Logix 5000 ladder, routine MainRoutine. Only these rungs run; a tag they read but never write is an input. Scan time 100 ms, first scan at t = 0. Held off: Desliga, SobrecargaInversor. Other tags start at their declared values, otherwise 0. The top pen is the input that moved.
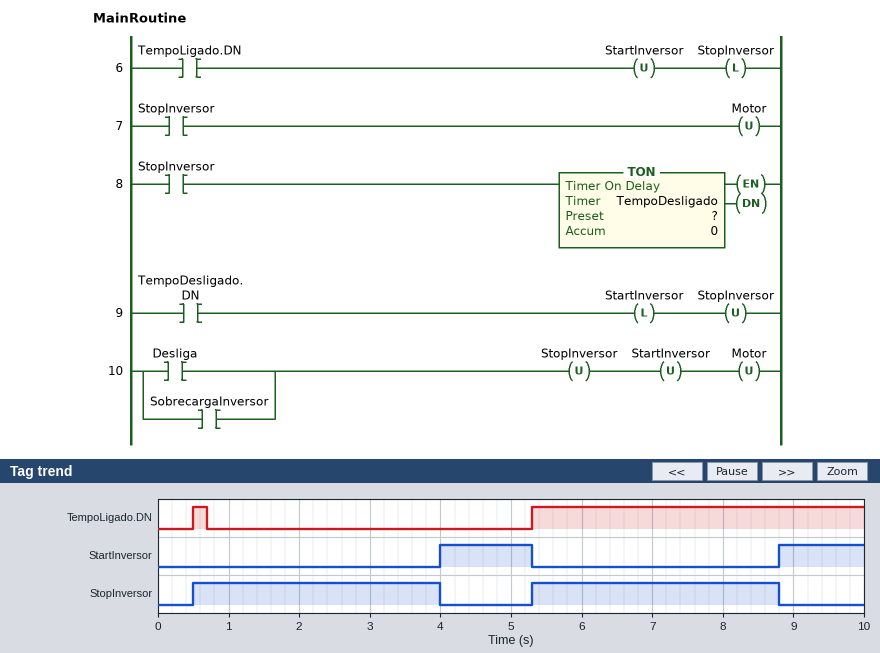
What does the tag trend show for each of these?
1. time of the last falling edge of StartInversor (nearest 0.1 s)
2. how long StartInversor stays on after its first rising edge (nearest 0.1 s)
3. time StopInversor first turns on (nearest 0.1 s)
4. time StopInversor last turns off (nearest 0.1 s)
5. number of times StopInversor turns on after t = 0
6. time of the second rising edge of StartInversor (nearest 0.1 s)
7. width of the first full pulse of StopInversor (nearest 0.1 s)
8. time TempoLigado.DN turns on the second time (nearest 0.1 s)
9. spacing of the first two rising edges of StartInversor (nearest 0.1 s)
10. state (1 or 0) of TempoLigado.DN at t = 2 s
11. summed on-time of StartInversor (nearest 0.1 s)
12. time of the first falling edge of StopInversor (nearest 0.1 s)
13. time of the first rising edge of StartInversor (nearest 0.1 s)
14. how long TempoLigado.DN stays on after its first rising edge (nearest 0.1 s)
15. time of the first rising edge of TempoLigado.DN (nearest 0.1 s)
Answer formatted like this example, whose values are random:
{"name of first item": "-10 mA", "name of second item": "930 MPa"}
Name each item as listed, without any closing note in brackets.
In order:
{"time of the last falling edge of StartInversor": "5.3 s", "how long StartInversor stays on after its first rising edge": "1.3 s", "time StopInversor first turns on": "0.5 s", "time StopInversor last turns off": "8.8 s", "number of times StopInversor turns on after t = 0": "2", "time of the second rising edge of StartInversor": "8.8 s", "width of the first full pulse of StopInversor": "3.5 s", "time TempoLigado.DN turns on the second time": "5.3 s", "spacing of the first two rising edges of StartInversor": "4.8 s", "state (1 or 0) of TempoLigado.DN at t = 2 s": "0", "summed on-time of StartInversor": "2.5 s", "time of the first falling edge of StopInversor": "4.0 s", "time of the first rising edge of StartInversor": "4.0 s", "how long TempoLigado.DN stays on after its first rising edge": "0.2 s", "time of the first rising edge of TempoLigado.DN": "0.5 s"}
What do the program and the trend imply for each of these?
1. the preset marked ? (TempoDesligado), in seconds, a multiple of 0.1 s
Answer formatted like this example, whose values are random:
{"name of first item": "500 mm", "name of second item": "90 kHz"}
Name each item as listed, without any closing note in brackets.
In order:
{"the preset marked ? (TempoDesligado), in seconds, a multiple of 0.1 s": "3.5 s"}
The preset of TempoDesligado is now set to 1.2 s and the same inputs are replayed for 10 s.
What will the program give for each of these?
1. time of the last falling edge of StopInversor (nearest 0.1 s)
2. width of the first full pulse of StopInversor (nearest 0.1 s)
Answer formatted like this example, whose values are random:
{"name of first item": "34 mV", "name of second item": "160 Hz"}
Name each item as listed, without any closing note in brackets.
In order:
{"time of the last falling edge of StopInversor": "6.5 s", "width of the first full pulse of StopInversor": "1.2 s"}
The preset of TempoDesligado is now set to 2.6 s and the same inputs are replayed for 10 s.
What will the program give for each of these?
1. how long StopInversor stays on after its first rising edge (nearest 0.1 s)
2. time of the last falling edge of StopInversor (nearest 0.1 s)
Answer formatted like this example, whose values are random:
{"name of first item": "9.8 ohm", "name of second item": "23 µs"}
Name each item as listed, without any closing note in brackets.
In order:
{"how long StopInversor stays on after its first rising edge": "2.6 s", "time of the last falling edge of StopInversor": "7.9 s"}
